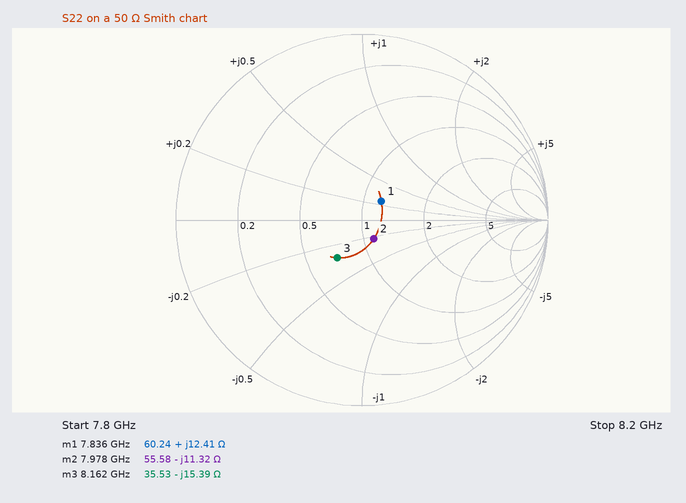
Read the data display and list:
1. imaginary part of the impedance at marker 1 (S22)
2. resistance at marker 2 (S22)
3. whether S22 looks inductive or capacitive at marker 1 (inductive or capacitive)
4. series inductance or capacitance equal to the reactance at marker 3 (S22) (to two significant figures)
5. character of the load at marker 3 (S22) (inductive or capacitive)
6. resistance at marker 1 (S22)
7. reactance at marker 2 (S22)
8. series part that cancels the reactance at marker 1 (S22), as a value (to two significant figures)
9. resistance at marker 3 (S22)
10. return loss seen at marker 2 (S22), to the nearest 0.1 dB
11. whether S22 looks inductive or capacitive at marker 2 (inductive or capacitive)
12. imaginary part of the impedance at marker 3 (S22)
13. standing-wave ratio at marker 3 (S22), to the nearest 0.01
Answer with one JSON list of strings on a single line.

["+12.41 Ω", "55.58 Ω", "inductive", "1.3 pF", "capacitive", "60.24 Ω", "-11.32 Ω", "1.6 pF", "35.53 Ω", "18.5 dB", "capacitive", "-15.39 Ω", "1.64"]
